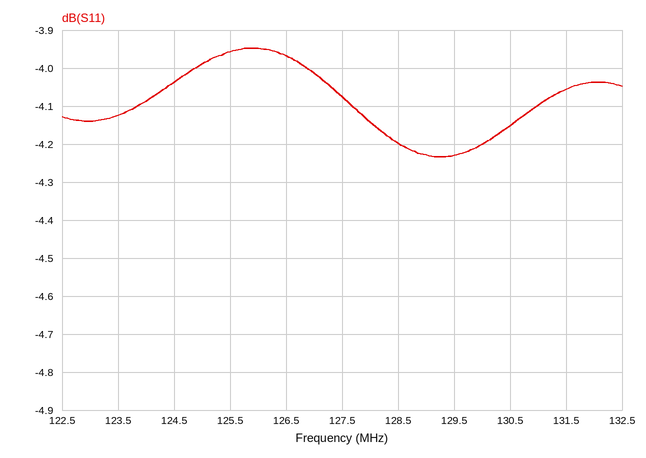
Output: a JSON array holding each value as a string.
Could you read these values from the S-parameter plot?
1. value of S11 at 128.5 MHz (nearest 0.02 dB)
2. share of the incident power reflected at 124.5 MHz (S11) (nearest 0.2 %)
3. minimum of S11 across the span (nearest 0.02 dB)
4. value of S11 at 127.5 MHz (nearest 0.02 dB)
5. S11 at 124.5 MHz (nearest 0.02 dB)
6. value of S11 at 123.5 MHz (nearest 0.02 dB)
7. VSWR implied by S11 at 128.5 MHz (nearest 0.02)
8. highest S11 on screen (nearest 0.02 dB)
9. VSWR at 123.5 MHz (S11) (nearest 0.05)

["-4.20 dB", "39.4 %", "-4.24 dB", "-4.08 dB", "-4.04 dB", "-4.12 dB", "4.22", "-3.94 dB", "4.30"]
